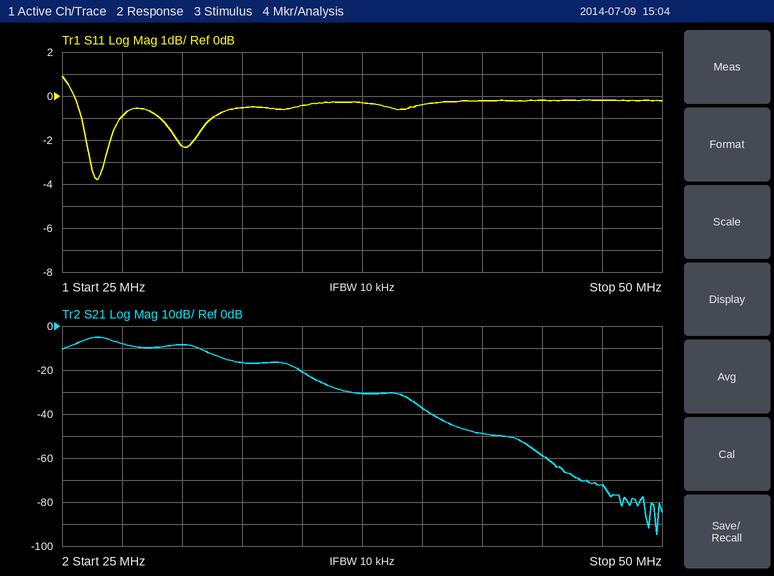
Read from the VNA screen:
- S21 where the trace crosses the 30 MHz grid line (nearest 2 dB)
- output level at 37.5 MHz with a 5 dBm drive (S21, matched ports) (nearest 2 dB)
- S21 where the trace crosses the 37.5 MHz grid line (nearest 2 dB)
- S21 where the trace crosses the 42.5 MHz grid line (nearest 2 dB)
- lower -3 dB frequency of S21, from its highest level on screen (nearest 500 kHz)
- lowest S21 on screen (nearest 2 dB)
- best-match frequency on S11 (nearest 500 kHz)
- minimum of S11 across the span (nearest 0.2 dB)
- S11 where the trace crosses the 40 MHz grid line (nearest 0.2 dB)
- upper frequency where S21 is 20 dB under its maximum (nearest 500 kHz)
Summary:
-8 dB
-26 dBm
-30 dB
-48 dB
25.5 MHz
-94 dB
26.5 MHz
-3.8 dB
-0.4 dB
35.5 MHz
